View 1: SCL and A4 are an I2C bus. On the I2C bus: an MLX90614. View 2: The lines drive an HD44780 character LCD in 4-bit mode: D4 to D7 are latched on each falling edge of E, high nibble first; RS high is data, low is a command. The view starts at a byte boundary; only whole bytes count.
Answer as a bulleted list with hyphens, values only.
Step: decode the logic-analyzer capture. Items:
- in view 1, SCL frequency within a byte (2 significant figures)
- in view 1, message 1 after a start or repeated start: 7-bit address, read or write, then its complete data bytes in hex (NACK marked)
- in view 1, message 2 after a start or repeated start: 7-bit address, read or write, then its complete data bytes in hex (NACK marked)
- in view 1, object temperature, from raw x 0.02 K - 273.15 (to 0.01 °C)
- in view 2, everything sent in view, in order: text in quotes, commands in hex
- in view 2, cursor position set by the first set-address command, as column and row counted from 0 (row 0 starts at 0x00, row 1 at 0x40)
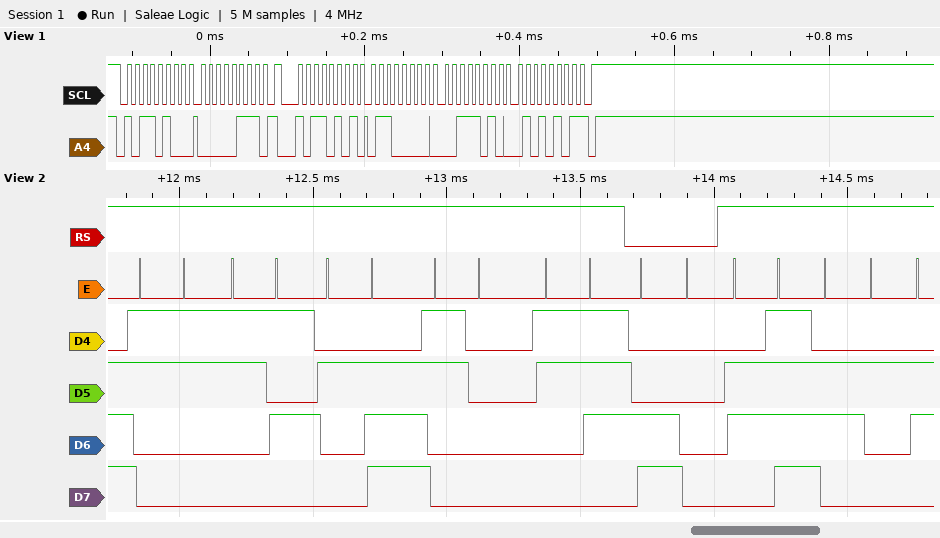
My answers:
- 100 kHz
- 0x5A write: 07
- 0x5A read: 60 3A 55 NACK
- 25.73 °C
- "35.07" 0xC0 "ob"
- column 0, row 1
